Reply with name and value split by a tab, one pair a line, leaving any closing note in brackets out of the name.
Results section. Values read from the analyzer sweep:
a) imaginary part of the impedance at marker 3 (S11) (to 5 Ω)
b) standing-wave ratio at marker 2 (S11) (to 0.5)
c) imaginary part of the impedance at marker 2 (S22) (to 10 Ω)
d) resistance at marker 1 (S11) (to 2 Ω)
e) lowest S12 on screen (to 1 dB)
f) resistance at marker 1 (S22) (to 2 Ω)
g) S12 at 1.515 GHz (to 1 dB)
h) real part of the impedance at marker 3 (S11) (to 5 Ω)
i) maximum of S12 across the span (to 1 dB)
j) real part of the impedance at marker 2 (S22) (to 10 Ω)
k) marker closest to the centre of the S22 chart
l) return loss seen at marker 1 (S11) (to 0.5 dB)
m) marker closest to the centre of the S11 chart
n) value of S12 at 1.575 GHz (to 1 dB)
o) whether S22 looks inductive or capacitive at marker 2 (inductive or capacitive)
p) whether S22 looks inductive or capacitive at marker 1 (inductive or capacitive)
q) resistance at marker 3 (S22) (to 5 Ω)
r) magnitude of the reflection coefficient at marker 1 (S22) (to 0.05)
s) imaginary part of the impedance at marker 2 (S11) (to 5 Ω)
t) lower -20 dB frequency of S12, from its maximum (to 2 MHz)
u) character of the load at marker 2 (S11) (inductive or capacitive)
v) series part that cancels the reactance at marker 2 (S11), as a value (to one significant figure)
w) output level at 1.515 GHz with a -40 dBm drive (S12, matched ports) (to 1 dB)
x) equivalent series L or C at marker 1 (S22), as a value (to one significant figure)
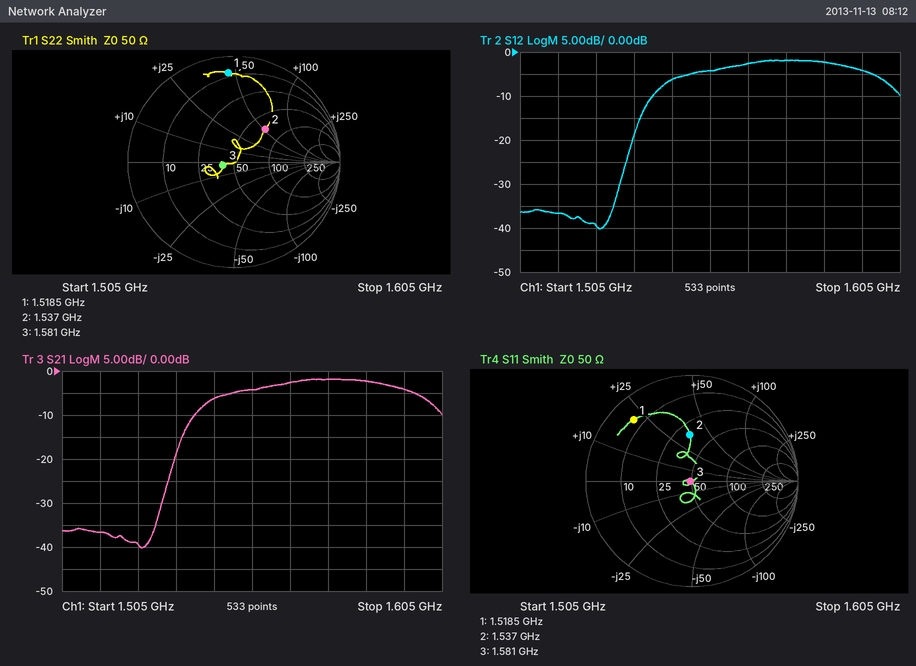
imaginary part of the impedance at marker 3 (S11)	0 Ω
standing-wave ratio at marker 2 (S11)	2.5
imaginary part of the impedance at marker 2 (S22)	+50 Ω
resistance at marker 1 (S11)	6 Ω
lowest S12 on screen	-40 dB
resistance at marker 1 (S22)	8 Ω
S12 at 1.515 GHz	-37 dB
real part of the impedance at marker 3 (S11)	50 Ω
maximum of S12 across the span	-2 dB
real part of the impedance at marker 2 (S22)	70 Ω
marker closest to the centre of the S22 chart	marker 3
return loss seen at marker 1 (S11)	2.0 dB
marker closest to the centre of the S11 chart	marker 3
value of S12 at 1.575 GHz	-2 dB
whether S22 looks inductive or capacitive at marker 2	inductive
whether S22 looks inductive or capacitive at marker 1	inductive
resistance at marker 3 (S22)	40 Ω
magnitude of the reflection coefficient at marker 1 (S22)	0.85
imaginary part of the impedance at marker 2 (S11)	+35 Ω
lower -20 dB frequency of S12, from its maximum	1.534 GHz
character of the load at marker 2 (S11)	inductive
series part that cancels the reactance at marker 2 (S11), as a value	3 pF
output level at 1.515 GHz with a -40 dBm drive (S12, matched ports)	-77 dBm
equivalent series L or C at marker 1 (S22), as a value	5 nH
